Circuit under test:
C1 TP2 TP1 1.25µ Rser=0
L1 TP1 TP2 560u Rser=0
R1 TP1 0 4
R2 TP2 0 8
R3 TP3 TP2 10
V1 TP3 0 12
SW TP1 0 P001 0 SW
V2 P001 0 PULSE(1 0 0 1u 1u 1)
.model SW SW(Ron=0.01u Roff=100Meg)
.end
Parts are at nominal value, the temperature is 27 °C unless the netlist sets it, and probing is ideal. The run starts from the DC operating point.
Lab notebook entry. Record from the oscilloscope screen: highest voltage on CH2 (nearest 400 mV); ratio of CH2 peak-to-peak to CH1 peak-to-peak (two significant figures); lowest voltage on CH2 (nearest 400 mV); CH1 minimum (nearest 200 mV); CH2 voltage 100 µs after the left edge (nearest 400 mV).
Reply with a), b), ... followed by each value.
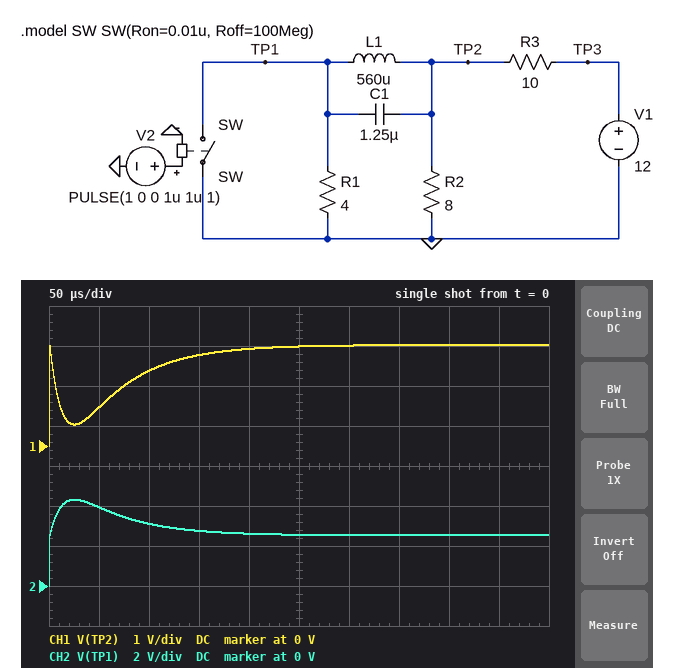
a) 4.4 V
b) 1.7
c) 0 V
d) 0 V
e) 3.2 V
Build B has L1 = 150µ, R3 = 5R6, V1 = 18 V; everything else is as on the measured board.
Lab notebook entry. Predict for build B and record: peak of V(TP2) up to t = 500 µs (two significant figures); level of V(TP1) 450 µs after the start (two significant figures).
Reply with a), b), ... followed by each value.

a) 5.9 V
b) 5.8 V
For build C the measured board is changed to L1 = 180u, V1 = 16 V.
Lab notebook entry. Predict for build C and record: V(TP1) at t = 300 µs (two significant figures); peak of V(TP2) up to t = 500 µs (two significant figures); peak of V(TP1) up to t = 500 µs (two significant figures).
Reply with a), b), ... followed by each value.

a) 3.4 V
b) 3.5 V
c) 5.3 V
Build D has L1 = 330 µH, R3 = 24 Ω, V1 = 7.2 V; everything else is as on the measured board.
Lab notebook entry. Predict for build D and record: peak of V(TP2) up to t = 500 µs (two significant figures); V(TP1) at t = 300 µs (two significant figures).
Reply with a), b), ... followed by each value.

a) 730 mV
b) 720 mV
